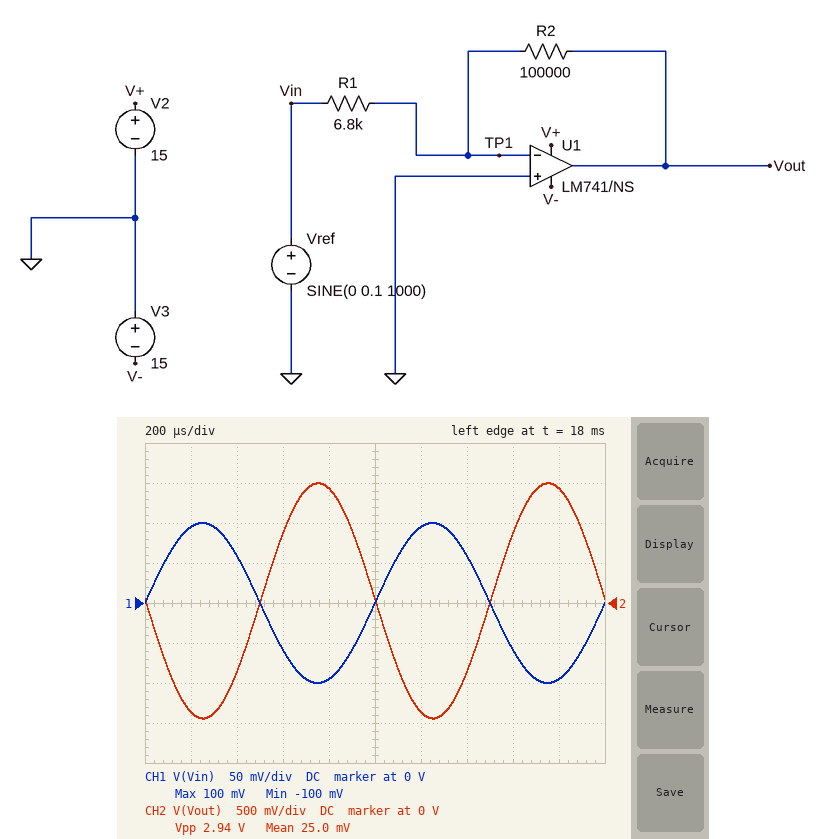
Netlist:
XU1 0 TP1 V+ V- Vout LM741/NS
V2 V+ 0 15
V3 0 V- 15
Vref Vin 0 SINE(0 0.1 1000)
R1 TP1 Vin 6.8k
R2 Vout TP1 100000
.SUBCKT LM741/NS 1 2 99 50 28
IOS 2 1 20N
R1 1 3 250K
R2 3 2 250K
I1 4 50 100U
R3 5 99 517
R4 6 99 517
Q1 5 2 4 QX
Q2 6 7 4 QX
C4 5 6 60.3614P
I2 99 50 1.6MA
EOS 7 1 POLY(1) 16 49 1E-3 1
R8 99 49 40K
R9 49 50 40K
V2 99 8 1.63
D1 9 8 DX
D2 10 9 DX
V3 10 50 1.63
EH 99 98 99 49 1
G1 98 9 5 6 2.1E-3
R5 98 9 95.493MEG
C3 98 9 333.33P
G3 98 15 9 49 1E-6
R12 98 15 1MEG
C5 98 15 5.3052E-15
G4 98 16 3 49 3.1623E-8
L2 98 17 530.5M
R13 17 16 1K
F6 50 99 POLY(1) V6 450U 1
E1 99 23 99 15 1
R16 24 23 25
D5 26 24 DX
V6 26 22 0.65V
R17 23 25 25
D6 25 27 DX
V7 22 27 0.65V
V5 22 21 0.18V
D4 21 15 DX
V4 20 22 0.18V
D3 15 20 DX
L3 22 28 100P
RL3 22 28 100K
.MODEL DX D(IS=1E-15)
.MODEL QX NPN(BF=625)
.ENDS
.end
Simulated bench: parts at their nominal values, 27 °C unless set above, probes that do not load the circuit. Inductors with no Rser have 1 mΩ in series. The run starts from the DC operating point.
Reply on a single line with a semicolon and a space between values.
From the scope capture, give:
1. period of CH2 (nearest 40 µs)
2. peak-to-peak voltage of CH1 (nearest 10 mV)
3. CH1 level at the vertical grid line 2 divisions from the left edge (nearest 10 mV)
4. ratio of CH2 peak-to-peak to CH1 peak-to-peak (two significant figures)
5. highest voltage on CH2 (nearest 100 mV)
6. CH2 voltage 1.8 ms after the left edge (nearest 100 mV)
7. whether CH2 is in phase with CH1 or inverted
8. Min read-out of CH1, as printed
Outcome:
1.00 ms; 200 mV; 60 mV; 15; 1.5 V; 1.4 V; inverted; -100 mV
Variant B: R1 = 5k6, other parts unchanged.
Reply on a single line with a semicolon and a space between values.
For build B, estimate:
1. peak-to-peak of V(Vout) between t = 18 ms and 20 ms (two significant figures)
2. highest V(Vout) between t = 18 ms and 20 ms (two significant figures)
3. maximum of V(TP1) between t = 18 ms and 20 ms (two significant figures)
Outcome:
3.6 V; 1.8 V; 2.8 mV
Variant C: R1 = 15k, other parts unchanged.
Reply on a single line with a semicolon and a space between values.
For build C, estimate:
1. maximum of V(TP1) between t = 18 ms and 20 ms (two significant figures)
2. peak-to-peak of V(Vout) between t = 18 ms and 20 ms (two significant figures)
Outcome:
1.7 mV; 1.3 V
